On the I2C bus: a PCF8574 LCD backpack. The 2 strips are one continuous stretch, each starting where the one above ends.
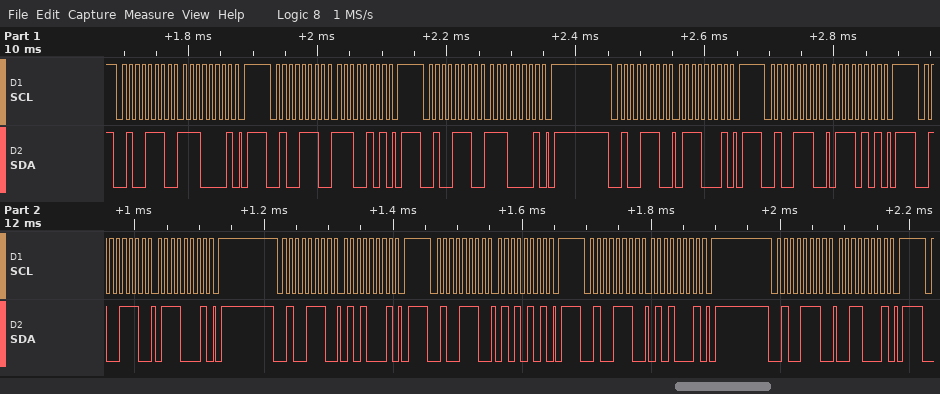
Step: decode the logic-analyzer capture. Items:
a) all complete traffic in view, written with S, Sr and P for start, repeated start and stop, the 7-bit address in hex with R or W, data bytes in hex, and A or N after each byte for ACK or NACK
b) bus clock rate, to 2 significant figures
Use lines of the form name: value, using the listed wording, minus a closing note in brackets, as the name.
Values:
all complete traffic in view, written with S, Sr and P for start, repeated start and stop, the 7-bit address in hex with R or W, data bytes in hex, and A or N after each byte for ACK or NACK: S 27W A E1 A P S 27W A E5 A P S 27W A E1 A P S 27W A 71 A P S 27W A 75 A P S 27W A 71 A P S 27W A 51 A P S 27W A 55 A P S 27W A 51 A P S 27W A 31 A P
bus clock rate, to 2 significant figures: 100 kHz
